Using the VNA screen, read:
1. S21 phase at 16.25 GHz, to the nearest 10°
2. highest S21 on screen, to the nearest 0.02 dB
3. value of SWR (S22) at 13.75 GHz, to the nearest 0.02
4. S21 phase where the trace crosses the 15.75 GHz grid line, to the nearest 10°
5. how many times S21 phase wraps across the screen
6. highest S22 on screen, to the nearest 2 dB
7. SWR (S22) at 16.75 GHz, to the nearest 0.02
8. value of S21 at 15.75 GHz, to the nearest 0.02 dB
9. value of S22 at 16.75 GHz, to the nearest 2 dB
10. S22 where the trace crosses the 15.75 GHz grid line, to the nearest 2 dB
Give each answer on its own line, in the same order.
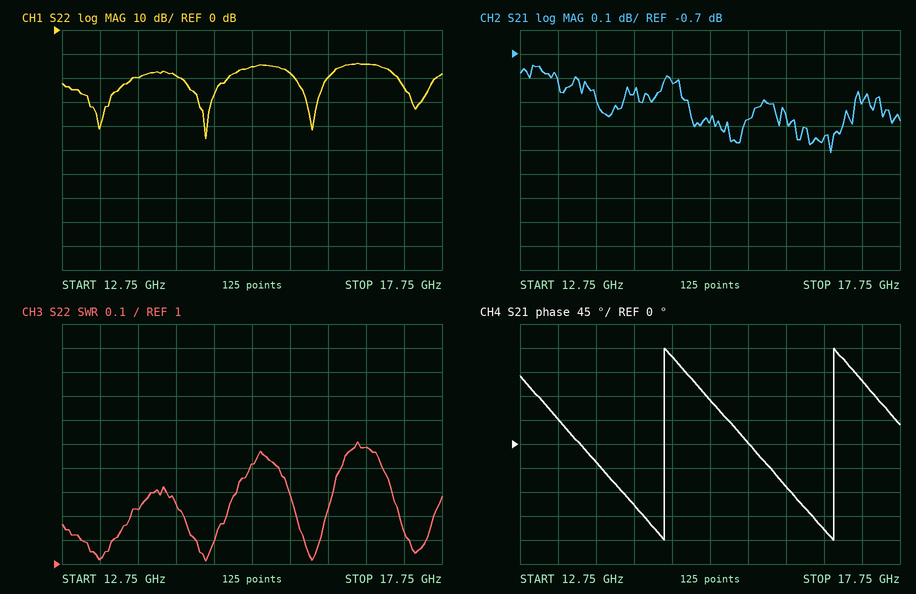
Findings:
-80°
-0.74 dB
1.22
0°
2
-14 dB
1.48
-0.98 dB
-14 dB
-18 dB
